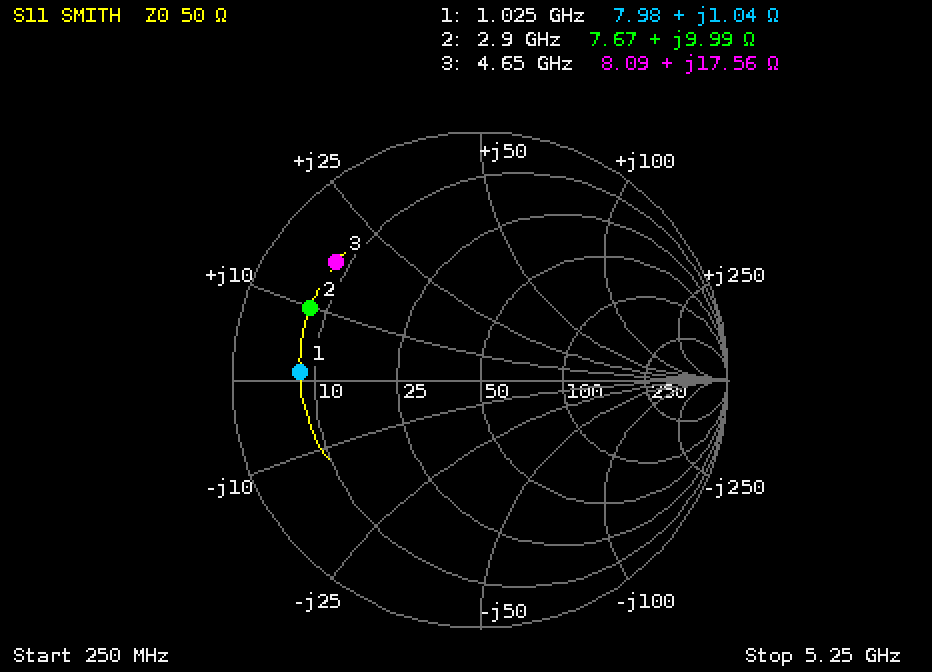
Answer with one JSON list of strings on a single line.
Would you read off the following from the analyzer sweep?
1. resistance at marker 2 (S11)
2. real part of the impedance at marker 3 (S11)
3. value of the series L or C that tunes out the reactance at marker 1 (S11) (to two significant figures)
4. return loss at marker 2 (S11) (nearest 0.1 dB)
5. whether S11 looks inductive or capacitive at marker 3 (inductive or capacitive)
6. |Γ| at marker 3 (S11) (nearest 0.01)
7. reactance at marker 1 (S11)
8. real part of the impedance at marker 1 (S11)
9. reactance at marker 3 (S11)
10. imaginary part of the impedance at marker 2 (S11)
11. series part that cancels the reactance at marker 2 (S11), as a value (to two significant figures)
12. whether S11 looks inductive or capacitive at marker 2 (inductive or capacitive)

["7.67 Ω", "8.09 Ω", "150 pF", "2.6 dB", "inductive", "0.75", "+1.04 Ω", "7.98 Ω", "+17.56 Ω", "+9.99 Ω", "5.5 pF", "inductive"]
